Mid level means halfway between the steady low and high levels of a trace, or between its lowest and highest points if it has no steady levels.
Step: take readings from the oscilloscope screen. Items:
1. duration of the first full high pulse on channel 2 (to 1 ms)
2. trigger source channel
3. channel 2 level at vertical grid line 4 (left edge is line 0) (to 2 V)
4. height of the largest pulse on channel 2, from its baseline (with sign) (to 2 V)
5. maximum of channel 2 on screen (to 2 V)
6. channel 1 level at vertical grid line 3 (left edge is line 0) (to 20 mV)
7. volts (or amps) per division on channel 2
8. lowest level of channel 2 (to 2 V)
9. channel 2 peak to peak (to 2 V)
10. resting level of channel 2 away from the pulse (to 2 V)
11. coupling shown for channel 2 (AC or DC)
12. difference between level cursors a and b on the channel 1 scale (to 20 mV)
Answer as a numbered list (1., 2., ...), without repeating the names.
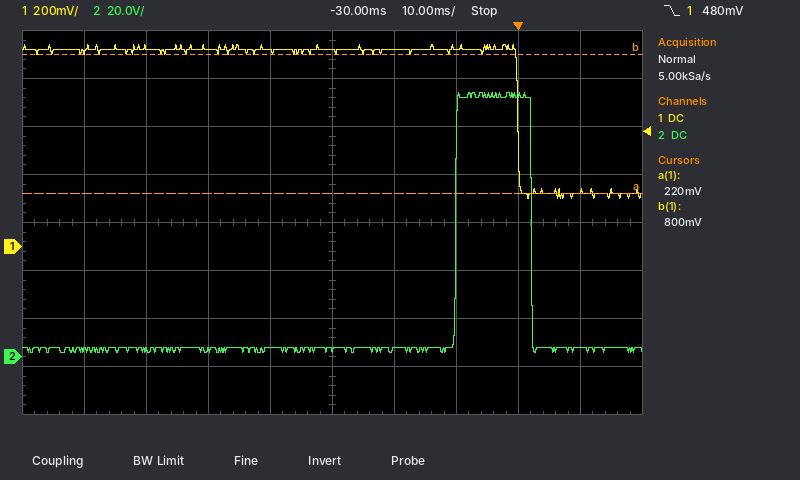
1. 12 ms
2. channel 1
3. 4 V
4. +106 V
5. 110 V
6. 820 mV
7. 20 V
8. 2 V
9. 108 V
10. 4 V
11. DC
12. 580 mV
